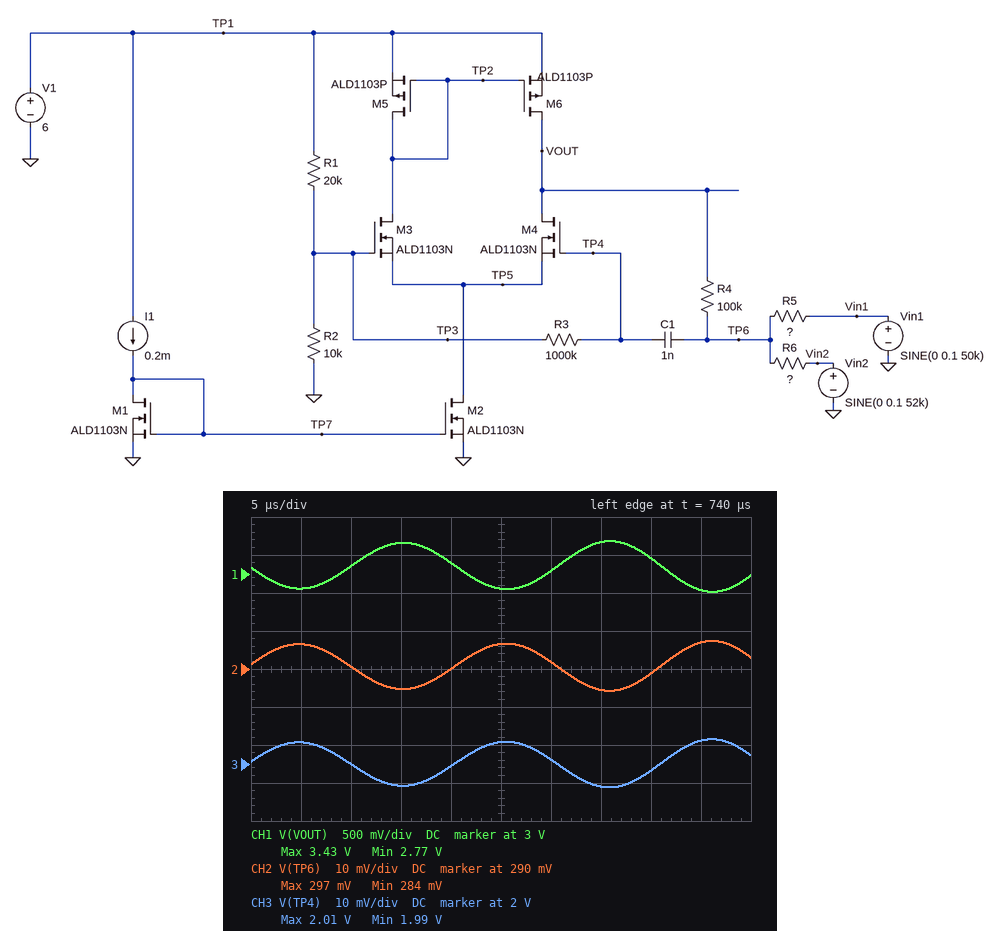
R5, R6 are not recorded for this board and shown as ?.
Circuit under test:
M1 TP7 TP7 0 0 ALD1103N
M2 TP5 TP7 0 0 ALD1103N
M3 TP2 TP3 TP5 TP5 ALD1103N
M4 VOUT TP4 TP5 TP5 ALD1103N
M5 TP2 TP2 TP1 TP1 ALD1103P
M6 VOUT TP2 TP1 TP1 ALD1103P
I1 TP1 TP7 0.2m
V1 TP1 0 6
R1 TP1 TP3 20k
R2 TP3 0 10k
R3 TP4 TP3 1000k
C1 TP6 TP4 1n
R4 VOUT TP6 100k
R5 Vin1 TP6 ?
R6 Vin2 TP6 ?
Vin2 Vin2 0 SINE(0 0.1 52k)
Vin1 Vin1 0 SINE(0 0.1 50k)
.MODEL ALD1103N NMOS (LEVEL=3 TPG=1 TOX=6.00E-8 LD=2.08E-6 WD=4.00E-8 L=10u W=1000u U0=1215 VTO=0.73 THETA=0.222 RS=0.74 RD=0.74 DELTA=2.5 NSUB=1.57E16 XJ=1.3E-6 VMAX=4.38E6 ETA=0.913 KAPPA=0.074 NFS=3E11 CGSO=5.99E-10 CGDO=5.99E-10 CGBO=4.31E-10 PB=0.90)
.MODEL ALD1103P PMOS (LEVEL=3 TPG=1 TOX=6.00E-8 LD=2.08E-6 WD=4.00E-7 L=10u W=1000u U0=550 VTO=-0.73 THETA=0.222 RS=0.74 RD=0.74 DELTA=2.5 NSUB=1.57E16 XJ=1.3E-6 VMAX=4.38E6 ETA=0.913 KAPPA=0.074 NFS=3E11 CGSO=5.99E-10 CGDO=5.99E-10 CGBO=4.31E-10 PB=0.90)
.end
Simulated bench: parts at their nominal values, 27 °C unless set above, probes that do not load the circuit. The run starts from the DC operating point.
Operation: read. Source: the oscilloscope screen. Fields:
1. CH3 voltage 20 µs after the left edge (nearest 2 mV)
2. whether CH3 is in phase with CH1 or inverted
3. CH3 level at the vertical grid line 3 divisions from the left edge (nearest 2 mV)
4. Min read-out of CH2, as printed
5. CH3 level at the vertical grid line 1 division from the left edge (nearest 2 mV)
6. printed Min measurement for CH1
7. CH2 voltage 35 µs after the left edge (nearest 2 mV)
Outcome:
2.000 V
inverted
1.994 V
284 mV
2.006 V
2.77 V
284 mV
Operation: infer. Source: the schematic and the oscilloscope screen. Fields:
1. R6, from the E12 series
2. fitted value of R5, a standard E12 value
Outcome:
33 kΩ
15 kΩ
